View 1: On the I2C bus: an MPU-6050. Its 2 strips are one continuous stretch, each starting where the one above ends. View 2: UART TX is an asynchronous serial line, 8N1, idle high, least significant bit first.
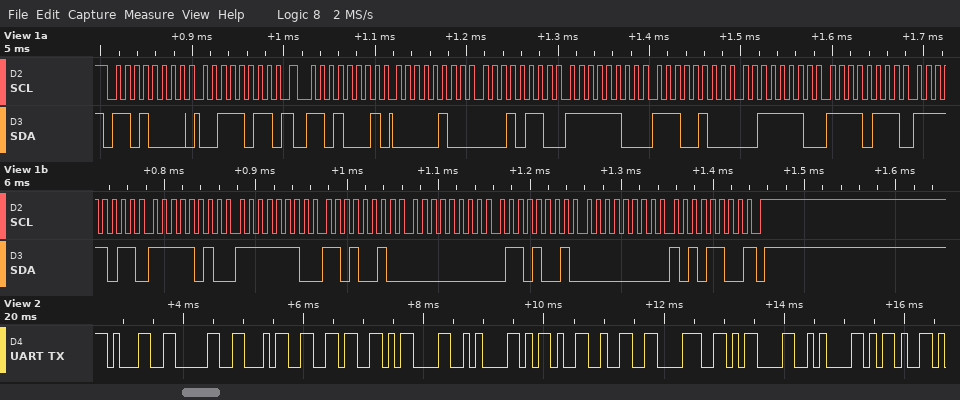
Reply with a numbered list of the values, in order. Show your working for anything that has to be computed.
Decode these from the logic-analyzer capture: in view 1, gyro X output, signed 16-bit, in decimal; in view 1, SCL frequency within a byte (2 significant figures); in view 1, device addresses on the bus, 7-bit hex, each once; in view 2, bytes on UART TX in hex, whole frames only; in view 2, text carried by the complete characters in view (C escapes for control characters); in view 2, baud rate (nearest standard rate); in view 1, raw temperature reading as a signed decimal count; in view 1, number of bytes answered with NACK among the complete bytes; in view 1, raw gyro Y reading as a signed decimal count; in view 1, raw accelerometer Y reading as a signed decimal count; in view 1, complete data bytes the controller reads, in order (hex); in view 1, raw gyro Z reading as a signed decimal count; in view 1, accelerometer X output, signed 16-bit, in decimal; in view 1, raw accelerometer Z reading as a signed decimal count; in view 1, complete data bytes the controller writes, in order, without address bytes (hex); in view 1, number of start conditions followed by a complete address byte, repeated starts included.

1. 0xFED2 = -302
2. 100 kHz
3. 0x68
4. 0x31 0x30 0x34 0x36 0x0D 0x0A 0x2D 0x32 0x38 0x0D 0x0A 0x2D
5. "1046\r\n-28\r\n-"
6. 9600 baud
7. 0xFBFA = -1030
8. 1
9. 0x0069 = 105
10. 0xFCE4 = -796
11. 04 16 FC E4 3E F7 FB FA FE D2 00 69 00 AC
12. 0x00AC = 172
13. 0x0416 = 1046
14. 0x3EF7 = 16119
15. 3B
16. 2
